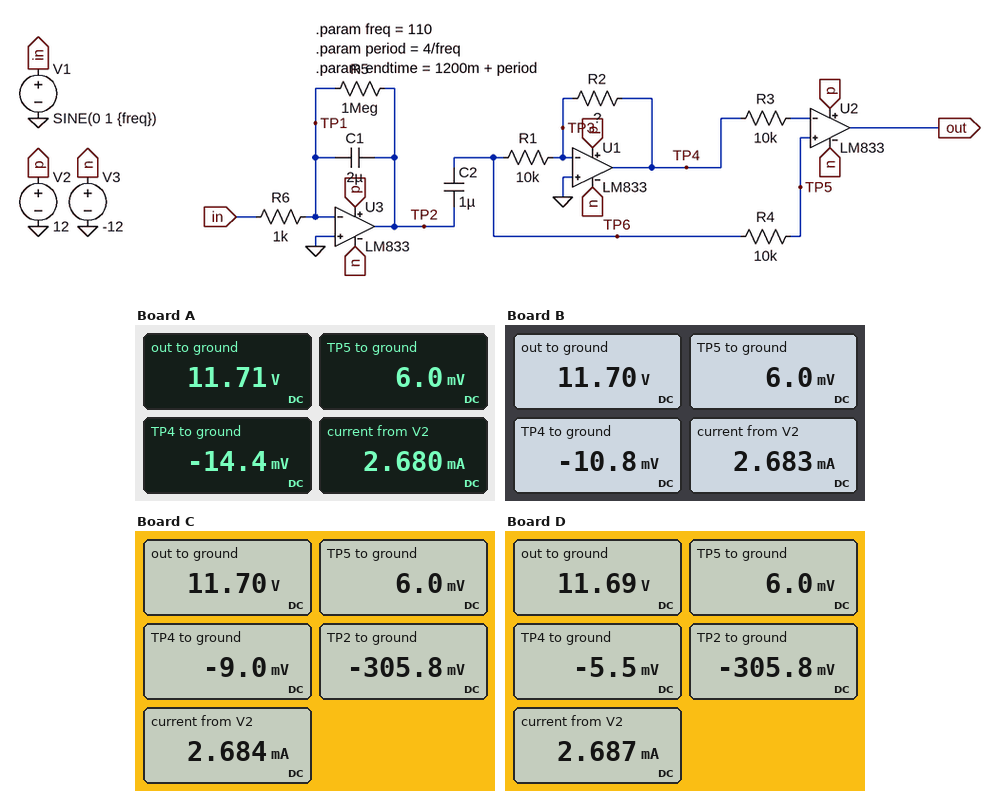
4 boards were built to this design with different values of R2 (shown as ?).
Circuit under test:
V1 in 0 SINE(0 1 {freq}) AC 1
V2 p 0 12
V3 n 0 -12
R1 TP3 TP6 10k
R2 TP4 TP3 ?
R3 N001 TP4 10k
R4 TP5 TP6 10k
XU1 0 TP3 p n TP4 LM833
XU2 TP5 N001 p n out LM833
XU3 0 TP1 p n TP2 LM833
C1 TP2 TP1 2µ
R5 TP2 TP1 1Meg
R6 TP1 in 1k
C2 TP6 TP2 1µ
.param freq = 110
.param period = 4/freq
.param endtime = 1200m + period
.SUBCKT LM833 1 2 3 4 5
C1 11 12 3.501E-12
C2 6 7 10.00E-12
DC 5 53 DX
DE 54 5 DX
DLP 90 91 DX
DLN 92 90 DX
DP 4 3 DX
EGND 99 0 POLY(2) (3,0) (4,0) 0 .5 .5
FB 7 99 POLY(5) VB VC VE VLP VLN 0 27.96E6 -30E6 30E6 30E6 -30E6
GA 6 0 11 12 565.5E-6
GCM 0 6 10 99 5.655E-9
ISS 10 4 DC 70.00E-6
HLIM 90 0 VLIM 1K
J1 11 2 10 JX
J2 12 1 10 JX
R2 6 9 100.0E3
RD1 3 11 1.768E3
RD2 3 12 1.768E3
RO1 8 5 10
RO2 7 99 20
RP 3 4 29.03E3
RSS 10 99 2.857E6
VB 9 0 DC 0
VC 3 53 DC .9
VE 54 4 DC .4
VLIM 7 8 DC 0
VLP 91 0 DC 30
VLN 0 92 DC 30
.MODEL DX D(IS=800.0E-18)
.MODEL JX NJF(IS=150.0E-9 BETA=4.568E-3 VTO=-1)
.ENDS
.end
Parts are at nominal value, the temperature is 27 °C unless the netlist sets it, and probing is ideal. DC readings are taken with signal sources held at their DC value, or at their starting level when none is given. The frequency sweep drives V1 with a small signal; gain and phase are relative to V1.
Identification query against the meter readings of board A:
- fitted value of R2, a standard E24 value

24 kΩ
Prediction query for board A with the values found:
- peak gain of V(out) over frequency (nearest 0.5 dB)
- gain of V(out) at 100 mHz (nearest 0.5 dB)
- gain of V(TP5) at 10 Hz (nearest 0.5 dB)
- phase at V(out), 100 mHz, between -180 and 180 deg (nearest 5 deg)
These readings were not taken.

28.0 dB
26.0 dB
12.5 dB
-140 deg
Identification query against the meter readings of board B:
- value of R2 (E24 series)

18 kΩ
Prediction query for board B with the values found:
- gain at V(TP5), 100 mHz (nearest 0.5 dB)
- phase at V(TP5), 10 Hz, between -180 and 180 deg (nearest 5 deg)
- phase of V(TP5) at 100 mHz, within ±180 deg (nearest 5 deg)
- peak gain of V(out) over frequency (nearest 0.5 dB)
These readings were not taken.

12.0 dB
150 deg
-140 deg
28.5 dB
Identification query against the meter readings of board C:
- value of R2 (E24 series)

15 kΩ
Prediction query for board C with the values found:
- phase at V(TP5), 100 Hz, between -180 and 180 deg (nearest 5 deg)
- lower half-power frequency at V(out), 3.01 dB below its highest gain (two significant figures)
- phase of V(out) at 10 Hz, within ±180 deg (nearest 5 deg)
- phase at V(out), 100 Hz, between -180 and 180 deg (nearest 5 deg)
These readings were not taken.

100 deg
79 mHz
150 deg
100 deg
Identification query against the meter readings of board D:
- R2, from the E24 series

9.1 kΩ
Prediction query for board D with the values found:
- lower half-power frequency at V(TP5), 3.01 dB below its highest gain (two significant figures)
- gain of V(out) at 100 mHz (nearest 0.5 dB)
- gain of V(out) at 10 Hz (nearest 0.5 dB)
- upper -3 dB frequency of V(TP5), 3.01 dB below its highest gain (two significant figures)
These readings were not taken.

79 mHz
27.0 dB
28.0 dB
16 Hz
